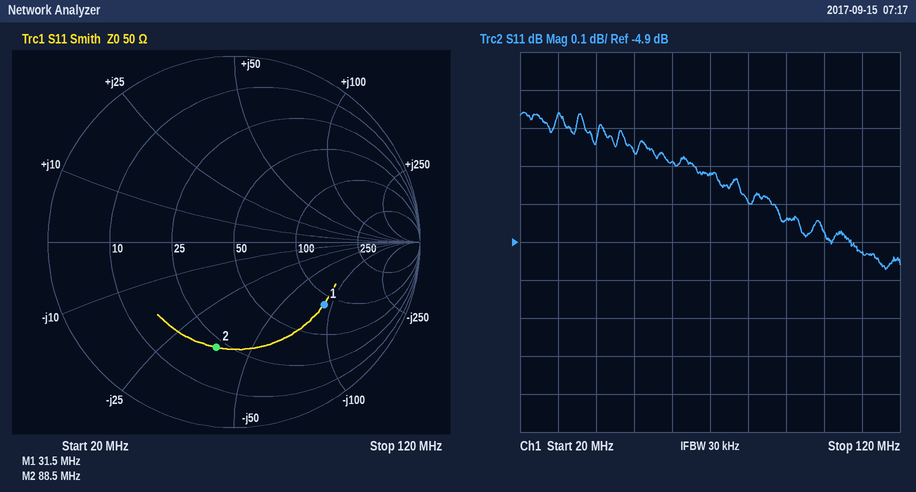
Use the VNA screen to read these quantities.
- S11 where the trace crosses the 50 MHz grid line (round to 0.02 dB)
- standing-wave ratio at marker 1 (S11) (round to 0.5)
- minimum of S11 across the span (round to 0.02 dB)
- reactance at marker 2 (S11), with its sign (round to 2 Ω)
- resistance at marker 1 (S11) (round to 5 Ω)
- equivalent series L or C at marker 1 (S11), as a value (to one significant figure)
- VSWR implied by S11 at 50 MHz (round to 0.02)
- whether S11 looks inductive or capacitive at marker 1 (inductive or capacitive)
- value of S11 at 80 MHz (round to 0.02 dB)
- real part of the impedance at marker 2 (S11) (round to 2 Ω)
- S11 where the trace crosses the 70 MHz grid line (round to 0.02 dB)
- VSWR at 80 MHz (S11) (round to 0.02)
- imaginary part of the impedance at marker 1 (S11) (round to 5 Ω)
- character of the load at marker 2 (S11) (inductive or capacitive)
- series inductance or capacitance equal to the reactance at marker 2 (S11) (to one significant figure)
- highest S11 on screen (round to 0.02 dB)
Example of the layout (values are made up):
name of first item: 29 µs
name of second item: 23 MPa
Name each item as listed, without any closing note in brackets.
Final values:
S11 where the trace crosses the 50 MHz grid line: -4.66 dB
standing-wave ratio at marker 1 (S11): 4.0
minimum of S11 across the span: -4.98 dB
reactance at marker 2 (S11), with its sign: -38 Ω
resistance at marker 1 (S11): 85 Ω
equivalent series L or C at marker 1 (S11), as a value: 60 pF
VSWR implied by S11 at 50 MHz: 3.82
whether S11 looks inductive or capacitive at marker 1: capacitive
value of S11 at 80 MHz: -4.80 dB
real part of the impedance at marker 2 (S11): 22 Ω
S11 where the trace crosses the 70 MHz grid line: -4.72 dB
VSWR at 80 MHz (S11): 3.72
imaginary part of the impedance at marker 1 (S11): -90 Ω
character of the load at marker 2 (S11): capacitive
series inductance or capacitance equal to the reactance at marker 2 (S11): 50 pF
highest S11 on screen: -4.56 dB
